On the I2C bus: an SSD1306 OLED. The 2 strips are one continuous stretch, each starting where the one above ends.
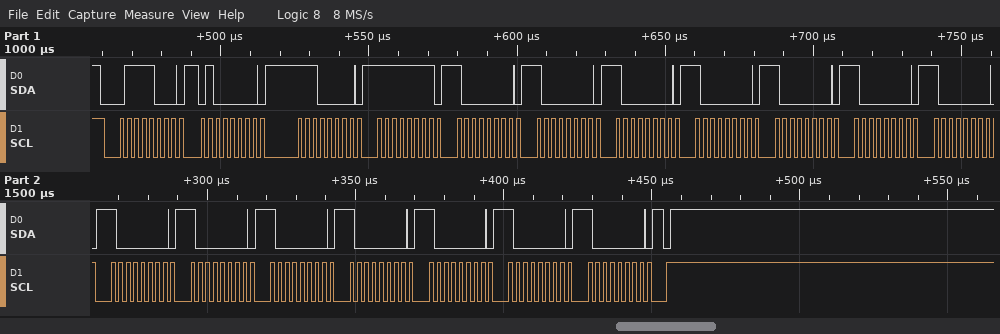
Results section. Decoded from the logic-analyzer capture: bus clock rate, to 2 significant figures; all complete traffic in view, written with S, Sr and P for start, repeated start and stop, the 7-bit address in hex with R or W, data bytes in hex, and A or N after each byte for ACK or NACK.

400 kHz
S 3CW A 40 A E0 A FF A 80 A 80 A 80 A 80 A 80 A 80 A 80 A 80 A 80 A 80 A 80 A 80 A 80 A 80 A P
